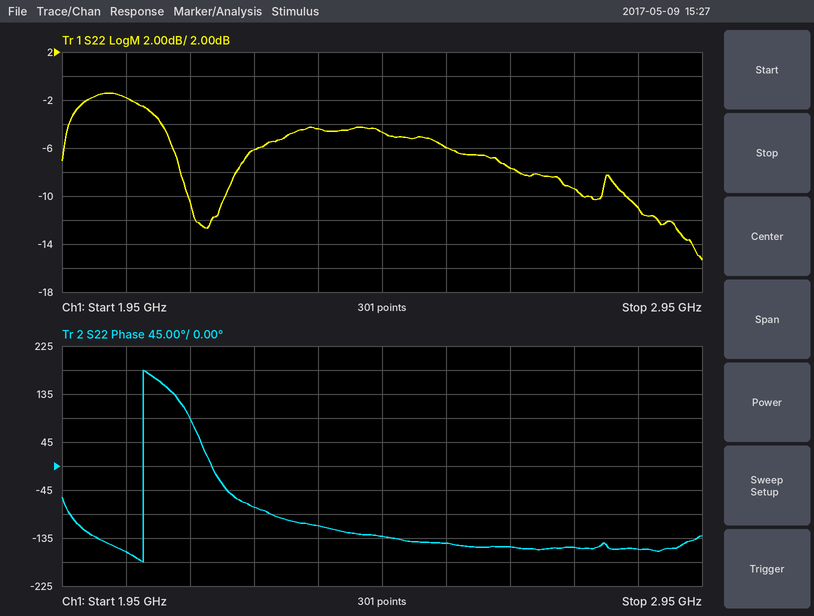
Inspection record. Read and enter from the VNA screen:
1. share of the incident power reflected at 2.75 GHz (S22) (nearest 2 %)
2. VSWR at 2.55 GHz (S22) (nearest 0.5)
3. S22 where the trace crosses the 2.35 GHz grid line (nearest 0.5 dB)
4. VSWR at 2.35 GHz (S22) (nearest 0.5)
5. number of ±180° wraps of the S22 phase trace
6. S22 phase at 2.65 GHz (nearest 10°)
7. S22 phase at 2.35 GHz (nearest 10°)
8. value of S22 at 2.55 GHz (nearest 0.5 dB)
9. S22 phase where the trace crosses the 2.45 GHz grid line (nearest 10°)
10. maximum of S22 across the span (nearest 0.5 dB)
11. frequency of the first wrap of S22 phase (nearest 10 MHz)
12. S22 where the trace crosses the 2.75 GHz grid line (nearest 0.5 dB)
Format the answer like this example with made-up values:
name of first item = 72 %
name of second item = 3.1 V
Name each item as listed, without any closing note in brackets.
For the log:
share of the incident power reflected at 2.75 GHz (S22) = 12 %
VSWR at 2.55 GHz (S22) = 3.0
S22 where the trace crosses the 2.35 GHz grid line = -4.5 dB
VSWR at 2.35 GHz (S22) = 4.0
number of ±180° wraps of the S22 phase trace = 1
S22 phase at 2.65 GHz = -150°
S22 phase at 2.35 GHz = -110°
value of S22 at 2.55 GHz = -6.0 dB
S22 phase where the trace crosses the 2.45 GHz grid line = -130°
maximum of S22 across the span = -1.5 dB
frequency of the first wrap of S22 phase = 2.08 GHz
S22 where the trace crosses the 2.75 GHz grid line = -9.5 dB
